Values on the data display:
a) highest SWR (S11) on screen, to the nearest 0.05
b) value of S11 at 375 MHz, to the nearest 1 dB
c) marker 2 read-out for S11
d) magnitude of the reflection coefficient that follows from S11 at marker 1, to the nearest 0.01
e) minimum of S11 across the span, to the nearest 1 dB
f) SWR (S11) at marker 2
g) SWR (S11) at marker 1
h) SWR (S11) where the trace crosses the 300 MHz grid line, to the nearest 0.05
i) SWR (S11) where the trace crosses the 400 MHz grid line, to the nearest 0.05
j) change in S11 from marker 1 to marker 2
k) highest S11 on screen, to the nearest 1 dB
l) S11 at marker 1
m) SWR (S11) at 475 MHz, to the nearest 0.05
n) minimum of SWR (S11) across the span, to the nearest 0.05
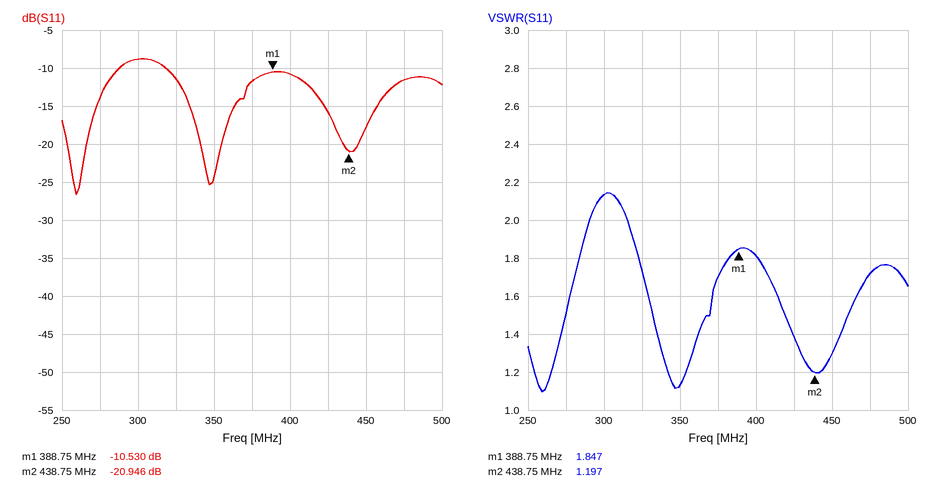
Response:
2.15
-12 dB
-20.946 dB
0.30
-27 dB
1.197
1.847
2.15
1.80
-10.416 dB
-9 dB
-10.530 dB
1.70
1.10
